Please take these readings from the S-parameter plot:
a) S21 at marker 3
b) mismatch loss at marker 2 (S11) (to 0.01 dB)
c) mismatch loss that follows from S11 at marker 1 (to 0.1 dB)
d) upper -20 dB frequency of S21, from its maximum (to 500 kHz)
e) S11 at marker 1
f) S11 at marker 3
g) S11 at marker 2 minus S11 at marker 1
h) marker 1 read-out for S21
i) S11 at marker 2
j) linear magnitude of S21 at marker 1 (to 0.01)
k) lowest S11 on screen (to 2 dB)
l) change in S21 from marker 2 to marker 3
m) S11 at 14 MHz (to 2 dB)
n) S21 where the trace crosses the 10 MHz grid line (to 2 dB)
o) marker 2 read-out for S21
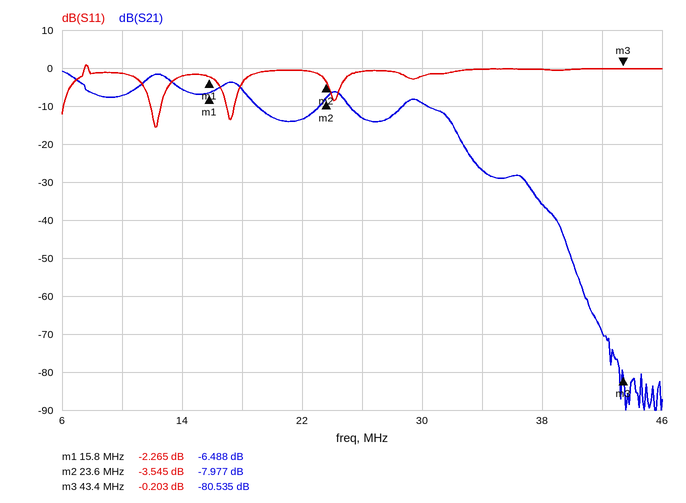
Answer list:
-80.535 dB
2.53 dB
3.9 dB
33.0 MHz
-2.265 dB
-0.203 dB
-1.280 dB
-6.488 dB
-3.545 dB
0.47
-16 dB
-72.558 dB
-2 dB
-8 dB
-7.977 dB
